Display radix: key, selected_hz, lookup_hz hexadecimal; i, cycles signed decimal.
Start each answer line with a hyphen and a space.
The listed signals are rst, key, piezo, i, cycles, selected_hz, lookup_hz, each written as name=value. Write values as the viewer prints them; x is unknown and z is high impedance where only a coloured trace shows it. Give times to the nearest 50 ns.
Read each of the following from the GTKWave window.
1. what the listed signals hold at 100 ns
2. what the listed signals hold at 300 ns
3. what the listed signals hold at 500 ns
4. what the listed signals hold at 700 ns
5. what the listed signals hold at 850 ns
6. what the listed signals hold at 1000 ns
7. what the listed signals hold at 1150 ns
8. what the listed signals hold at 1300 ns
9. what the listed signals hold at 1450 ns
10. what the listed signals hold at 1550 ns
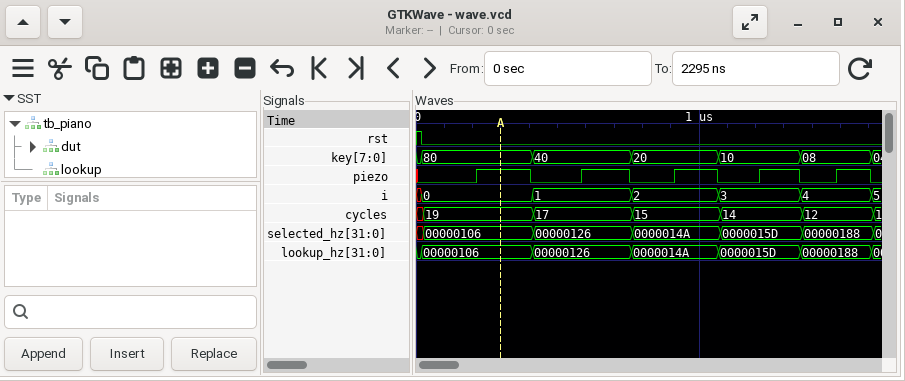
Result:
- rst=0, key=80, piezo=0, i=0, cycles=19, selected_hz=00000106, lookup_hz=00000106
- rst=0, key=80, piezo=1, i=0, cycles=19, selected_hz=00000106, lookup_hz=00000106
- rst=0, key=40, piezo=0, i=1, cycles=17, selected_hz=00000126, lookup_hz=00000126
- rst=0, key=40, piezo=1, i=1, cycles=17, selected_hz=00000126, lookup_hz=00000126
- rst=0, key=20, piezo=0, i=2, cycles=15, selected_hz=0000014A, lookup_hz=0000014A
- rst=0, key=20, piezo=1, i=2, cycles=15, selected_hz=0000014A, lookup_hz=0000014A
- rst=0, key=10, piezo=0, i=3, cycles=14, selected_hz=0000015D, lookup_hz=0000015D
- rst=0, key=10, piezo=1, i=3, cycles=14, selected_hz=0000015D, lookup_hz=0000015D
- rst=0, key=08, piezo=0, i=4, cycles=12, selected_hz=00000188, lookup_hz=00000188
- rst=0, key=08, piezo=1, i=4, cycles=12, selected_hz=00000188, lookup_hz=00000188
